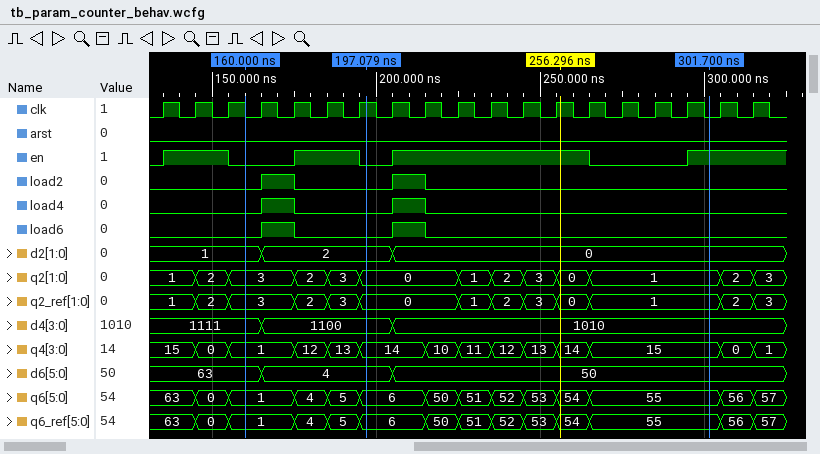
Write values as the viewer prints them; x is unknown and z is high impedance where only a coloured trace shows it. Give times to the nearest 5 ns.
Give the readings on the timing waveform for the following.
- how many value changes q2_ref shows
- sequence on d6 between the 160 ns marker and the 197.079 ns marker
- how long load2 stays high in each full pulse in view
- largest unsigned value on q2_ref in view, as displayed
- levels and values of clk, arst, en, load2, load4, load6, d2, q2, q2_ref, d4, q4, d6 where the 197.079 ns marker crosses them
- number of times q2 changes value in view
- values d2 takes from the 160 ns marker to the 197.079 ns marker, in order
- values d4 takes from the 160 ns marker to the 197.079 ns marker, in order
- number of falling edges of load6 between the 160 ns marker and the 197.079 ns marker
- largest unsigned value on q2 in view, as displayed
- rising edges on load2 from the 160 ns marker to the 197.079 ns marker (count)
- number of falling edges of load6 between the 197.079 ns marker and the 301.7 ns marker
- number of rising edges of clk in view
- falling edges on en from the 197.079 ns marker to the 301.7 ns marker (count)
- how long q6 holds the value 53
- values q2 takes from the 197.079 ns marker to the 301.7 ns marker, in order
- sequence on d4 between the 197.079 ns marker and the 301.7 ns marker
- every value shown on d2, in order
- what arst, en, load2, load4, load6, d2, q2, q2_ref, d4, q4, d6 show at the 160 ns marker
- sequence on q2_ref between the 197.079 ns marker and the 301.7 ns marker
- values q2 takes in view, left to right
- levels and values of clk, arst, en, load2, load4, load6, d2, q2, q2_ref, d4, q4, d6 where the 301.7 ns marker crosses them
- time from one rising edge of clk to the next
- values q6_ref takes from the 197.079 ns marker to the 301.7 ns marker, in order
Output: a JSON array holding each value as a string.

["12", "63, 4", "10 ns, 10 ns", "3", "clk=1, arst=0, en=0, load2=0, load4=0, load6=0, d2=2, q2=0, q2_ref=0, d4=1100, q4=14, d6=4", "12", "1, 2", "1111, 1100", "1", "3", "1", "1", "19", "1", "10 ns", "0, 1, 2, 3, 0, 1", "1100, 1010", "1, 2, 0", "arst=0, en=0, load2=0, load4=0, load6=0, d2=1, q2=3, q2_ref=3, d4=1111, q4=1, d6=63", "0, 1, 2, 3, 0, 1", "1, 2, 3, 2, 3, 0, 1, 2, 3, 0, 1, 2, 3", "clk=0, arst=0, en=1, load2=0, load4=0, load6=0, d2=0, q2=1, q2_ref=1, d4=1010, q4=15, d6=50", "10 ns", "6, 50, 51, 52, 53, 54, 55"]
